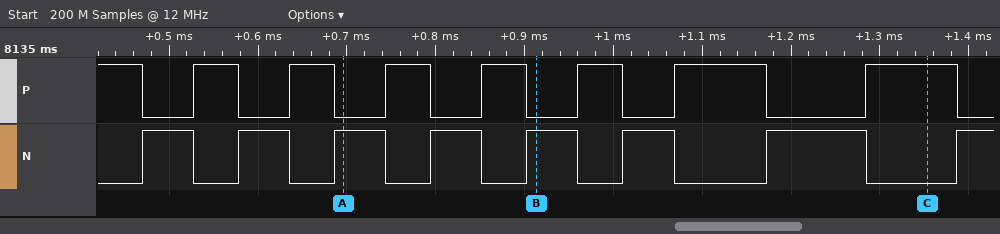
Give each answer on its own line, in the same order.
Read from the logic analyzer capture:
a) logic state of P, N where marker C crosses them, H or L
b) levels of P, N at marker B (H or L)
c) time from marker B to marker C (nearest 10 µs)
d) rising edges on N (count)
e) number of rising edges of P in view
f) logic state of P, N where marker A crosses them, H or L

P=H, N=L
P=L, N=H
440 µs
8
7
P=L, N=H
